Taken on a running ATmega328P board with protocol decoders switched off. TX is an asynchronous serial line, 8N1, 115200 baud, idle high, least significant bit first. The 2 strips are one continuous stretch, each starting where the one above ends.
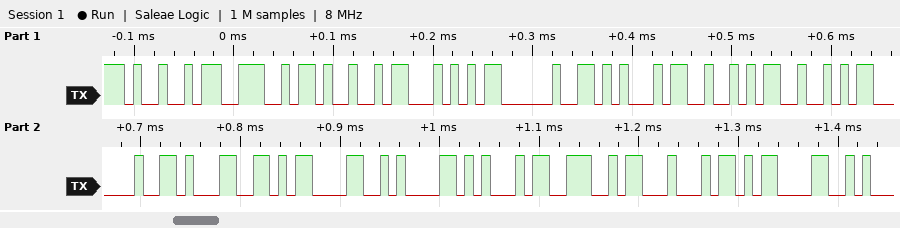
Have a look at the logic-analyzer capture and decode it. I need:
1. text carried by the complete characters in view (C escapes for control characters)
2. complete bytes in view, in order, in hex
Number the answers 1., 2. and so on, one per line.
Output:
1. "INIT ERR 1\r\nEND\r"
2. 49 4E 49 54 20 45 52 52 20 31 0D 0A 45 4E 44 0D
